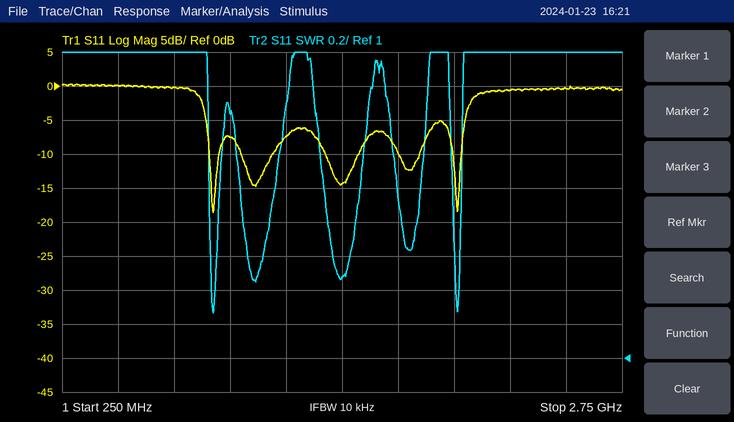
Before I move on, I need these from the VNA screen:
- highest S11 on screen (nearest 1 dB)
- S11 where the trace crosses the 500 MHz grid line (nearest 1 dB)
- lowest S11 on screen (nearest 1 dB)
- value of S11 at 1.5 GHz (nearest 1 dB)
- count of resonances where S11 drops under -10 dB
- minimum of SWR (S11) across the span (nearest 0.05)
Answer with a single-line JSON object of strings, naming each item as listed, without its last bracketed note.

{"highest S11 on screen": "0 dB", "S11 where the trace crosses the 500 MHz grid line": "0 dB", "lowest S11 on screen": "-19 dB", "value of S11 at 1.5 GHz": "-14 dB", "count of resonances where S11 drops under -10 dB": "5", "minimum of SWR (S11) across the span": "1.25"}
